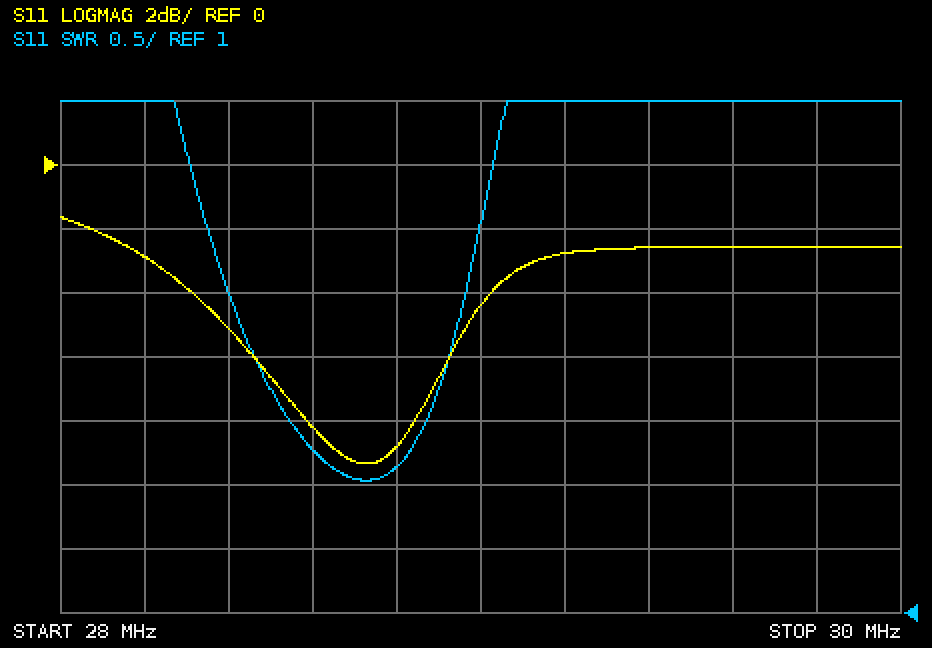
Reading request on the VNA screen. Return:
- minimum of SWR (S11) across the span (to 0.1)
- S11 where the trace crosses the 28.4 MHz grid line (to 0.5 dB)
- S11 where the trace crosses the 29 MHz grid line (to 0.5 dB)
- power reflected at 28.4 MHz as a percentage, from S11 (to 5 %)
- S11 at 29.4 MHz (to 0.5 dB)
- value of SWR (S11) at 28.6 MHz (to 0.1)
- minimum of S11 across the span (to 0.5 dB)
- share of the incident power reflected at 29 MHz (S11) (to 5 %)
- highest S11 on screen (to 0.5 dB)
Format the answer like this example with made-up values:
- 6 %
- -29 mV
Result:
- 2.0
- -5.0 dB
- -4.5 dB
- 30 %
- -2.5 dB
- 2.3
- -9.5 dB
- 35 %
- -1.5 dB
